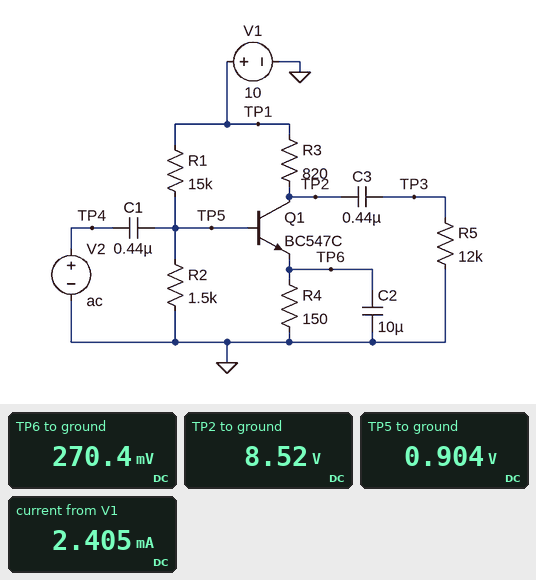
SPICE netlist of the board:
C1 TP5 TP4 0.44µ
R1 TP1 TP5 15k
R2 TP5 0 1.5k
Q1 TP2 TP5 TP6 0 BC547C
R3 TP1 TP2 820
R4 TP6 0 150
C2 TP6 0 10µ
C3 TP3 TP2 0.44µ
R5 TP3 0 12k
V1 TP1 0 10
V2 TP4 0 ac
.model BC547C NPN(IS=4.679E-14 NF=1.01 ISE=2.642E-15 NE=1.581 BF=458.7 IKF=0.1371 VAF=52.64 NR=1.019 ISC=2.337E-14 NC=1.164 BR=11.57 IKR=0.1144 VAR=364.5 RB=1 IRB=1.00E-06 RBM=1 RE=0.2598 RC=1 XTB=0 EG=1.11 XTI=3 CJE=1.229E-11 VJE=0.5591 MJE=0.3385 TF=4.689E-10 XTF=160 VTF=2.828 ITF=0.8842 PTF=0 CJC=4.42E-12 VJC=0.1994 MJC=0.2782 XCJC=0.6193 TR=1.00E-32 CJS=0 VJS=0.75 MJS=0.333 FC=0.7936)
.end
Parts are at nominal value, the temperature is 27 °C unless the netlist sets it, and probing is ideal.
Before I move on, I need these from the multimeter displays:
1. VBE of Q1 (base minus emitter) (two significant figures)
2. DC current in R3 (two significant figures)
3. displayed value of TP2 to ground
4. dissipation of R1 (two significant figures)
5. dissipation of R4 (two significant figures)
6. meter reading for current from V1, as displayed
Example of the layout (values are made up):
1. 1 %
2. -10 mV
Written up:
1. 630 mV
2. 1.8 mA
3. 8.52 V
4. 5.5 mW
5. 490 µW
6. 2.405 mA
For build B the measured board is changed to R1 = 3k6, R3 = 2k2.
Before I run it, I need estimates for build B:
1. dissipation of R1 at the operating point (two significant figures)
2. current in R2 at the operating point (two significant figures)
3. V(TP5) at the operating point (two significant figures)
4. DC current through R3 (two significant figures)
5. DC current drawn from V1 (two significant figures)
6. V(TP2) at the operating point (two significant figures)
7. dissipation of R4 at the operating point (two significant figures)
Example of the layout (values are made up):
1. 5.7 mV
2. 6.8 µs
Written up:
1. 20 mW
2. 1.0 mA
3. 1.5 V
4. 4.2 mA
5. 6.5 mA
6. 840 mV
7. 4.5 mW
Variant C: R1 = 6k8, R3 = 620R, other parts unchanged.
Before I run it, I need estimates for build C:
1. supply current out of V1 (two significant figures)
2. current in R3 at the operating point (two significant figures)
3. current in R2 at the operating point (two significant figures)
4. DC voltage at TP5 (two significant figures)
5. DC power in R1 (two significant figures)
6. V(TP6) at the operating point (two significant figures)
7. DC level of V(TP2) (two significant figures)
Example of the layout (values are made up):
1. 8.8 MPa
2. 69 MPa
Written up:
1. 8.6 mA
2. 7.4 mA
3. 1.2 mA
4. 1.8 V
5. 9.9 mW
6. 1.1 V
7. 5.4 V
